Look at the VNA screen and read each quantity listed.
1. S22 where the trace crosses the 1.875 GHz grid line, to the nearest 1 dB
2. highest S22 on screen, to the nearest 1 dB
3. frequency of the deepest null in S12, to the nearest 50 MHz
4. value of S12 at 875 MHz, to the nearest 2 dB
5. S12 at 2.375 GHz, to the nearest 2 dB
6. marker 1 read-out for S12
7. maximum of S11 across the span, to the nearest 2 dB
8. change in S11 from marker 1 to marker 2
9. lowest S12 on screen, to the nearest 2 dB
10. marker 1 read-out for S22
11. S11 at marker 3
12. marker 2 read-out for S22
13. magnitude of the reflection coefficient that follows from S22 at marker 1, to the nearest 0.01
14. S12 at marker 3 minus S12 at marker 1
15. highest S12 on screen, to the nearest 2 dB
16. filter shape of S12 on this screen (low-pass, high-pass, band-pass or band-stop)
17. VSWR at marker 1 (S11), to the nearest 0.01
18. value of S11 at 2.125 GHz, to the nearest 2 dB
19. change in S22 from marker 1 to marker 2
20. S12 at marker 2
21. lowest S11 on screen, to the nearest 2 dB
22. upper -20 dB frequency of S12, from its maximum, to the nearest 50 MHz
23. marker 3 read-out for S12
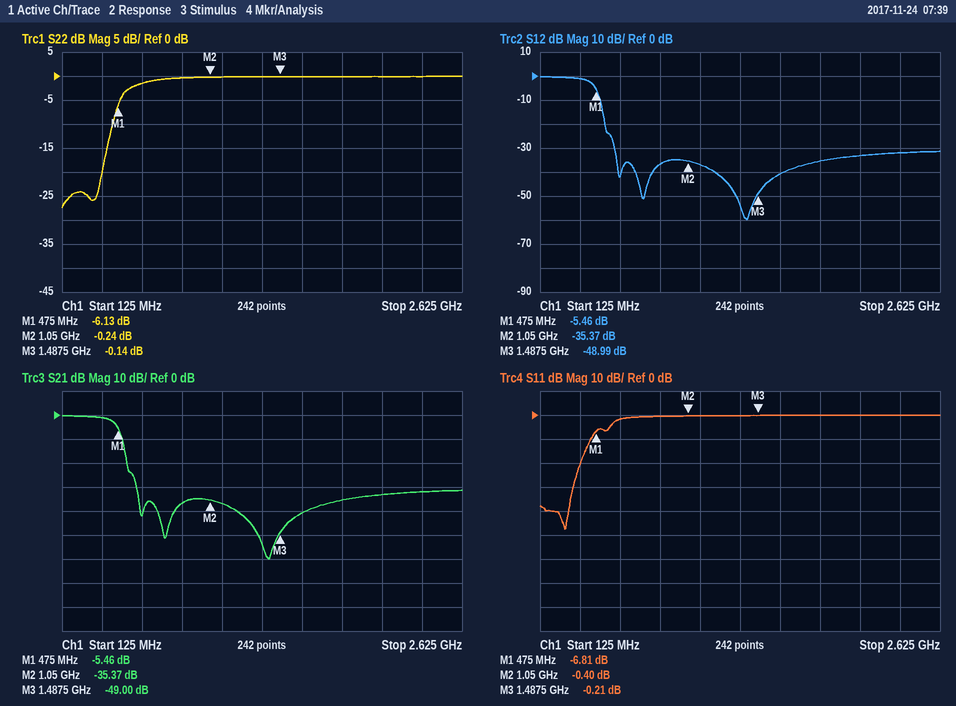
0 dB
0 dB
1.40 GHz
-36 dB
-32 dB
-5.46 dB
0 dB
6.41 dB
-60 dB
-6.13 dB
-0.21 dB
-0.24 dB
0.49
-43.53 dB
0 dB
low-pass
2.68
0 dB
5.89 dB
-35.37 dB
-48 dB
550 MHz
-48.99 dB
